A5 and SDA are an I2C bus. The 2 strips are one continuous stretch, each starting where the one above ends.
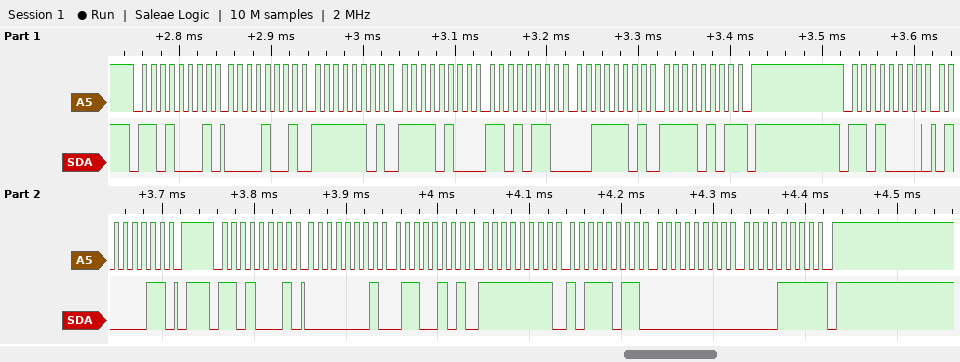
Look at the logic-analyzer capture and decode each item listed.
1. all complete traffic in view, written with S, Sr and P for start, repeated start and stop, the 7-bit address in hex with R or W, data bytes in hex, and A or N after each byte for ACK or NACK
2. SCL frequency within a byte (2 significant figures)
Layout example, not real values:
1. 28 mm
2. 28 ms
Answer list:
1. S 68R A 09 A FD A F4 A D6 A 3D A F5 N P S 68W A 43 A P S 68R A 01 A 65 A FF A BB A 00 A 0F N P
2. 100 kHz
